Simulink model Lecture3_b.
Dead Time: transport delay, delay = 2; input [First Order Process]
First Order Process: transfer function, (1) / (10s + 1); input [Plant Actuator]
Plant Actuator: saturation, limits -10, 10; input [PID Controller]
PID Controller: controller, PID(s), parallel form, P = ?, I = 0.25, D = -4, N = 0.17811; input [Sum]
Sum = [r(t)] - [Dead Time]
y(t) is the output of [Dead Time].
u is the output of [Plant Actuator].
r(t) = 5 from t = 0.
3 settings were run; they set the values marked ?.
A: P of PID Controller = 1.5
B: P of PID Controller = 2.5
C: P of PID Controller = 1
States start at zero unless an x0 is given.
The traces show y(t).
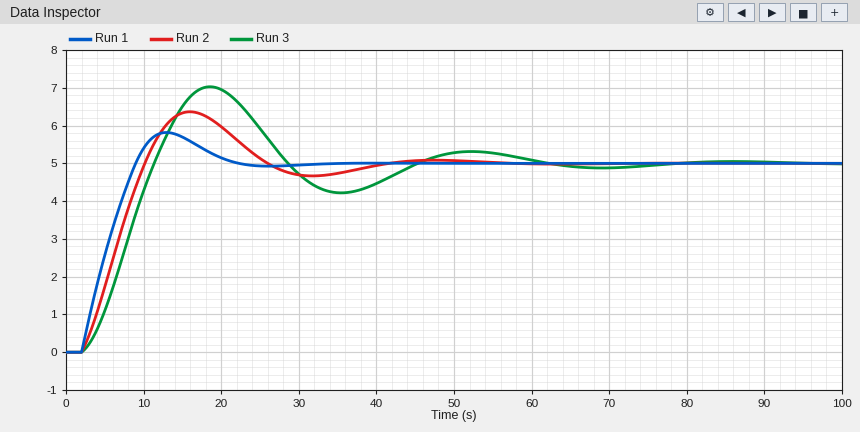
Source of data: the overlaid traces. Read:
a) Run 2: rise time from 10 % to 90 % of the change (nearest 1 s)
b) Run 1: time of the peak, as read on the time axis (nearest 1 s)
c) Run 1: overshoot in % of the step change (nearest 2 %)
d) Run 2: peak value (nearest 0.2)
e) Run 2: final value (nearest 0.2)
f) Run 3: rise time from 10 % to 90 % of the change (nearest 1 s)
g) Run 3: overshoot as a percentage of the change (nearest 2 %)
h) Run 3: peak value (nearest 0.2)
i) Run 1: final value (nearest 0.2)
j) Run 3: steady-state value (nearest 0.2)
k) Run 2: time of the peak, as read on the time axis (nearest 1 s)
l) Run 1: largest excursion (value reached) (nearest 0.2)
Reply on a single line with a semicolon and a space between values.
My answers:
6 s; 13 s; 16 %; 6.4; 5.0; 7 s; 40 %; 7.0; 5.0; 5.0; 16 s; 5.8
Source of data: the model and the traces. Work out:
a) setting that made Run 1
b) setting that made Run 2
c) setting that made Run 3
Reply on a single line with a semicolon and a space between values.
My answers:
B; A; C
